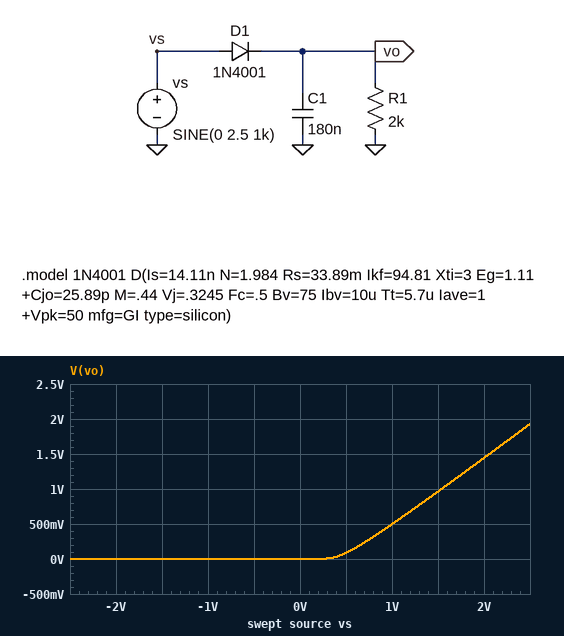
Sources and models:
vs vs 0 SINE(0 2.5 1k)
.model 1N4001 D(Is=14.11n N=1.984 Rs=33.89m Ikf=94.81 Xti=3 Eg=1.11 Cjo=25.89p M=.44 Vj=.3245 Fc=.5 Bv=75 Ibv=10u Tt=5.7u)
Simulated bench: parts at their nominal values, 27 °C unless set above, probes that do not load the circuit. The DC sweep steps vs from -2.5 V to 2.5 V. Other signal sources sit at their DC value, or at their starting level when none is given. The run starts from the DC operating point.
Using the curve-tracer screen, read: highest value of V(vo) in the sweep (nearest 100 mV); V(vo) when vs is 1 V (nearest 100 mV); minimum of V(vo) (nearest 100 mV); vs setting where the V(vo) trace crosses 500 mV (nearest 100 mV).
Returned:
1.9 V
500 mV
0 V
1.0 V
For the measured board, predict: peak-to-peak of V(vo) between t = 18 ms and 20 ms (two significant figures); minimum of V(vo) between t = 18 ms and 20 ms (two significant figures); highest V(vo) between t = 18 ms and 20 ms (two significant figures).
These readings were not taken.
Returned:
1.7 V
240 mV
1.9 V
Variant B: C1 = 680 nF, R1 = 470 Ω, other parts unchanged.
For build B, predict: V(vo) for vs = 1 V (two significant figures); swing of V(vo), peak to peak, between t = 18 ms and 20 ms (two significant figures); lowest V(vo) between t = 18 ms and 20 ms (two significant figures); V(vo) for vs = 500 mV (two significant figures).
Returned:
430 mV
1.7 V
180 mV
46 mV
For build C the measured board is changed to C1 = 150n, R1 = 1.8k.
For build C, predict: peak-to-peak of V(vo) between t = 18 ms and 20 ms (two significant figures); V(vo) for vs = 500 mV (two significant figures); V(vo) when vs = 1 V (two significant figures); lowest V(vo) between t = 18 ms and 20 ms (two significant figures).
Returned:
1.8 V
84 mV
490 mV
130 mV
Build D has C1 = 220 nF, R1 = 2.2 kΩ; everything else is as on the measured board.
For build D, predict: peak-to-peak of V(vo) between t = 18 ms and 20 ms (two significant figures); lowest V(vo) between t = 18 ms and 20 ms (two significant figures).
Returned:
1.5 V
400 mV
